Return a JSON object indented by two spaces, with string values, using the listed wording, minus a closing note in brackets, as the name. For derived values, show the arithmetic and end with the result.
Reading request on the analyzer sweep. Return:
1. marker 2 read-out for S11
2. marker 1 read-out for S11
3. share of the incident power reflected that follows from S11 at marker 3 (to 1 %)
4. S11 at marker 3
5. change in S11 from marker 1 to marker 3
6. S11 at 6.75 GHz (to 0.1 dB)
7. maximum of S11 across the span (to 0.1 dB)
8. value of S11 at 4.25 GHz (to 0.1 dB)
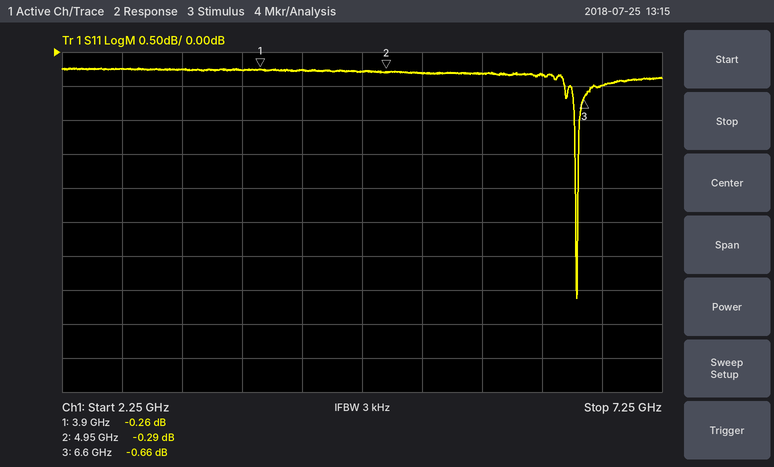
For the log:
{
  "marker 2 read-out for S11": "-0.29 dB",
  "marker 1 read-out for S11": "-0.26 dB",
  "share of the incident power reflected that follows from S11 at marker 3": "10^(-0.66/10) ≈ 86 %",
  "S11 at marker 3": "-0.66 dB",
  "change in S11 from marker 1 to marker 3": "-0.66 − (-0.26) = -0.40 dB",
  "S11 at 6.75 GHz": "-0.5 dB",
  "maximum of S11 across the span": "-0.2 dB",
  "value of S11 at 4.25 GHz": "-0.3 dB"
}
